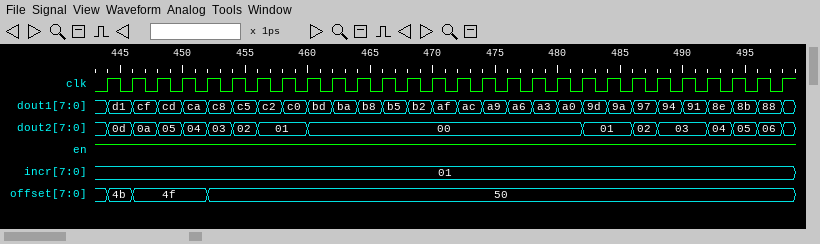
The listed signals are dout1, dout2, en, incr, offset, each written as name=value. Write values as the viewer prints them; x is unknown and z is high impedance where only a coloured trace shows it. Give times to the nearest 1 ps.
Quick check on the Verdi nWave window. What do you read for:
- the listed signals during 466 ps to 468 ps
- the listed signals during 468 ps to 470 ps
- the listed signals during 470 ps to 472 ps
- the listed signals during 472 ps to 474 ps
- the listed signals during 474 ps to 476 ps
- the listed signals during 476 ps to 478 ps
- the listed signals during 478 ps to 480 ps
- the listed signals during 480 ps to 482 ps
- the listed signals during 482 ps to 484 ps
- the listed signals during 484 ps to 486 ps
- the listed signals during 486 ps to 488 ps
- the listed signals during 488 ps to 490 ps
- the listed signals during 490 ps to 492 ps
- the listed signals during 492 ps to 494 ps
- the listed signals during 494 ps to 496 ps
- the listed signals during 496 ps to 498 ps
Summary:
dout1=b5, dout2=00, en=1, incr=01, offset=50
dout1=b2, dout2=00, en=1, incr=01, offset=50
dout1=af, dout2=00, en=1, incr=01, offset=50
dout1=ac, dout2=00, en=1, incr=01, offset=50
dout1=a9, dout2=00, en=1, incr=01, offset=50
dout1=a6, dout2=00, en=1, incr=01, offset=50
dout1=a3, dout2=00, en=1, incr=01, offset=50
dout1=a0, dout2=00, en=1, incr=01, offset=50
dout1=9d, dout2=01, en=1, incr=01, offset=50
dout1=9a, dout2=01, en=1, incr=01, offset=50
dout1=97, dout2=02, en=1, incr=01, offset=50
dout1=94, dout2=03, en=1, incr=01, offset=50
dout1=91, dout2=03, en=1, incr=01, offset=50
dout1=8e, dout2=04, en=1, incr=01, offset=50
dout1=8b, dout2=05, en=1, incr=01, offset=50
dout1=88, dout2=06, en=1, incr=01, offset=50
